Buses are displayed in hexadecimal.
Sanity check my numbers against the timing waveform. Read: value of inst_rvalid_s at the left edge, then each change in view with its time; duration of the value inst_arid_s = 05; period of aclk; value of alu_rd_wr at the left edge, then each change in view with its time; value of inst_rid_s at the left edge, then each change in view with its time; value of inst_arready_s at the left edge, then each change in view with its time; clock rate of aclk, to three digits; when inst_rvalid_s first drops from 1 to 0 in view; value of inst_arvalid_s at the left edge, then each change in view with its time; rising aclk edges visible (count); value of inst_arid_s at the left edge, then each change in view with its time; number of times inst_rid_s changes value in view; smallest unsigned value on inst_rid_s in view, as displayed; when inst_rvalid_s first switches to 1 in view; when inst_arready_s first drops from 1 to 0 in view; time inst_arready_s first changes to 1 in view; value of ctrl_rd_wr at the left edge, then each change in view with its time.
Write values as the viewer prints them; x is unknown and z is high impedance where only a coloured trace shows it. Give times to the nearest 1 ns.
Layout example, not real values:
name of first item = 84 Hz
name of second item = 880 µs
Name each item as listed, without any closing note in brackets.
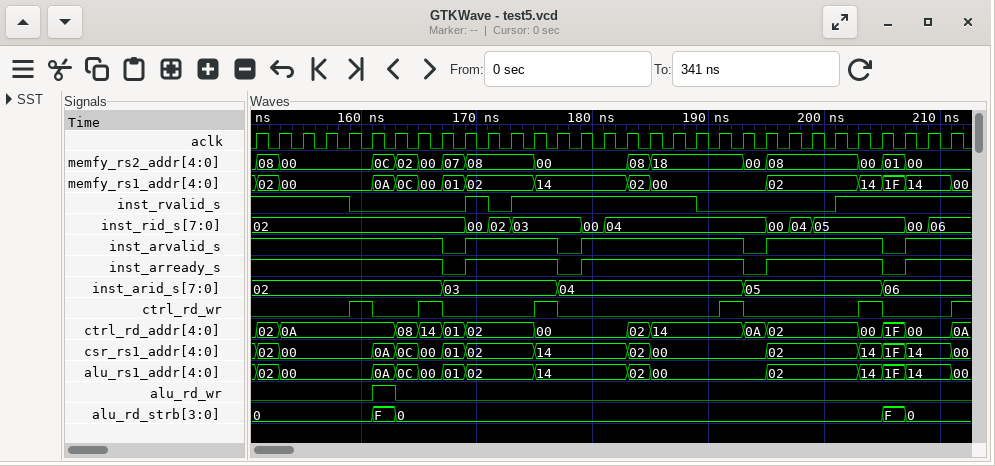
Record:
value of inst_rvalid_s at the left edge, then each change in view with its time = 1, 0 at 159 ns, 1 at 169 ns, 0 at 171 ns, 1 at 173 ns, 0 at 189 ns, 1 at 201 ns
duration of the value inst_arid_s = 05 = 12 ns
period of aclk = 2 ns
value of alu_rd_wr at the left edge, then each change in view with its time = 0, 1 at 161 ns, 0 at 163 ns
value of inst_rid_s at the left edge, then each change in view with its time = 02, 00 at 169 ns, 02 at 171 ns, 03 at 173 ns, 00 at 179 ns, 04 at 181 ns, 00 at 195 ns, 04 at 197 ns, 05 at 199 ns, 00 at 207 ns, 06 at 209 ns
value of inst_arready_s at the left edge, then each change in view with its time = 1, 0 at 167 ns, 1 at 169 ns, 0 at 177 ns, 1 at 179 ns, 0 at 193 ns, 1 at 195 ns, 0 at 205 ns, 1 at 207 ns
clock rate of aclk, to three digits = 500 MHz
when inst_rvalid_s first drops from 1 to 0 in view = 159 ns
value of inst_arvalid_s at the left edge, then each change in view with its time = 1, 0 at 167 ns, 1 at 169 ns, 0 at 177 ns, 1 at 179 ns, 0 at 193 ns, 1 at 195 ns, 0 at 205 ns, 1 at 207 ns
rising aclk edges visible = 31
value of inst_arid_s at the left edge, then each change in view with its time = 02, 03 at 167 ns, 04 at 177 ns, 05 at 193 ns, 06 at 205 ns
number of times inst_rid_s changes value in view = 10
smallest unsigned value on inst_rid_s in view, as displayed = 00
when inst_rvalid_s first switches to 1 in view = 169 ns
when inst_arready_s first drops from 1 to 0 in view = 167 ns
time inst_arready_s first changes to 1 in view = 169 ns
value of ctrl_rd_wr at the left edge, then each change in view with its time = 0, 1 at 159 ns, 0 at 161 ns, 1 at 165 ns, 0 at 167 ns, 1 at 175 ns, 0 at 177 ns, 1 at 191 ns, 0 at 193 ns, 1 at 203 ns, 0 at 205 ns, 1 at 211 ns
